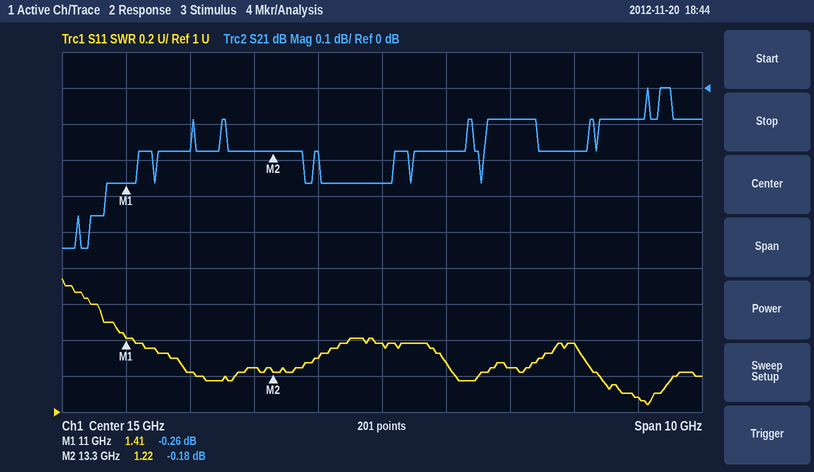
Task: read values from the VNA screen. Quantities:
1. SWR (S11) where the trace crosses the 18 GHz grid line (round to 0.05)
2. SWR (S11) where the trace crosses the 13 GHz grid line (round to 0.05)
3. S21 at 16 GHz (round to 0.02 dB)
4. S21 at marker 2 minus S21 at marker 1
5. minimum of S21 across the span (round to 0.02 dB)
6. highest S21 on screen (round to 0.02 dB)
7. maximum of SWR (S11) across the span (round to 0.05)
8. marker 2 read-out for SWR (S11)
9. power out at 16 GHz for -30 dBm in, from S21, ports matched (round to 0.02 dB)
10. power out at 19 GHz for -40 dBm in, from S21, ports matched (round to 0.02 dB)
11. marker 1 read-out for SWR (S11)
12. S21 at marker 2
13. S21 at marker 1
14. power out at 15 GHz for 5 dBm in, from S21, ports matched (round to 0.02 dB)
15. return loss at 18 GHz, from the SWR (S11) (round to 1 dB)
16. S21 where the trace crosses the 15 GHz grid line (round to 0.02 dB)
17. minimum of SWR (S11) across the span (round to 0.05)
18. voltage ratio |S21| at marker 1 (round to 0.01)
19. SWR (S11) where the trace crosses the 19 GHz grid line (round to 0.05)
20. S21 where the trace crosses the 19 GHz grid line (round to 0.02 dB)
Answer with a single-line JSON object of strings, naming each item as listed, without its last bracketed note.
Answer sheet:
{"SWR (S11) where the trace crosses the 18 GHz grid line": "1.40", "SWR (S11) where the trace crosses the 13 GHz grid line": "1.25", "S21 at 16 GHz": "-0.18 dB", "S21 at marker 2 minus S21 at marker 1": "0.08 dB", "minimum of S21 across the span": "-0.44 dB", "highest S21 on screen": "0.00 dB", "maximum of SWR (S11) across the span": "1.75", "marker 2 read-out for SWR": "1.22", "power out at 16 GHz for -30 dBm in, from S21, ports matched": "-30.18 dBm", "power out at 19 GHz for -40 dBm in, from S21, ports matched": "-40.08 dBm", "marker 1 read-out for SWR": "1.41", "S21 at marker 2": "-0.18 dB", "S21 at marker 1": "-0.26 dB", "power out at 15 GHz for 5 dBm in, from S21, ports matched": "4.74 dBm", "return loss at 18 GHz, from the SWR (S11)": "16 dB", "S21 where the trace crosses the 15 GHz grid line": "-0.26 dB", "minimum of SWR (S11) across the span": "1.05", "voltage ratio |S21| at marker 1": "0.97", "SWR (S11) where the trace crosses the 19 GHz grid line": "1.10", "S21 where the trace crosses the 19 GHz grid line": "-0.08 dB"}
